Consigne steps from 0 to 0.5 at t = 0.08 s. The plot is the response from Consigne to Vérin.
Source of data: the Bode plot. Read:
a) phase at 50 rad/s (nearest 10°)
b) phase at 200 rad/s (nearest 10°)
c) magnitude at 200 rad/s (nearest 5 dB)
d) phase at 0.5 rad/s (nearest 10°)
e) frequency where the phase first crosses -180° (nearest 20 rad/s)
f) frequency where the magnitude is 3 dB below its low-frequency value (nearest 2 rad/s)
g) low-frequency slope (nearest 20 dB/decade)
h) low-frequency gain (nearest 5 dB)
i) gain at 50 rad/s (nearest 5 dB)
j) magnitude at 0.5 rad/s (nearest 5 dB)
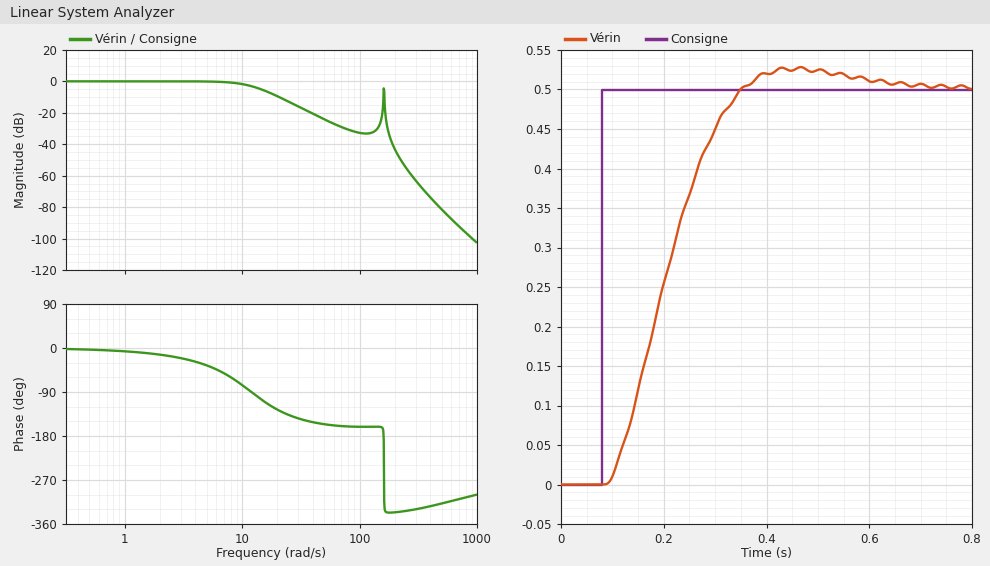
-160°
-340°
-45 dB
0°
160 rad/s
12 rad/s
0 dB/decade
0 dB
-25 dB
0 dB
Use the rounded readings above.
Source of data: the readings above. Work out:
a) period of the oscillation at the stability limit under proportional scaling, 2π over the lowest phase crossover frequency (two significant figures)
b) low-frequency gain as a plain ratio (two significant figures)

0.039 s
1.0
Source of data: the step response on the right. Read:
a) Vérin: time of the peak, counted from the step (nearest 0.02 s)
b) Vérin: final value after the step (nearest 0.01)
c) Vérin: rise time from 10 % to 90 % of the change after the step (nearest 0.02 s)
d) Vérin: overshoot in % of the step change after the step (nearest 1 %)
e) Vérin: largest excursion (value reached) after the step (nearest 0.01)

0.38 s
0.50
0.18 s
5 %
0.53
